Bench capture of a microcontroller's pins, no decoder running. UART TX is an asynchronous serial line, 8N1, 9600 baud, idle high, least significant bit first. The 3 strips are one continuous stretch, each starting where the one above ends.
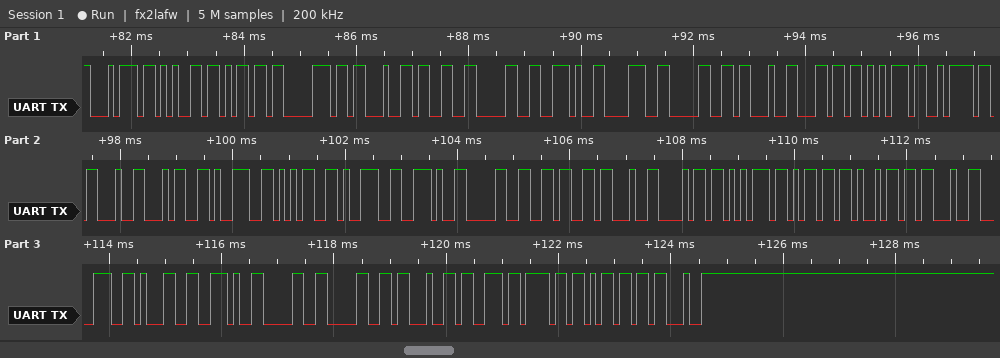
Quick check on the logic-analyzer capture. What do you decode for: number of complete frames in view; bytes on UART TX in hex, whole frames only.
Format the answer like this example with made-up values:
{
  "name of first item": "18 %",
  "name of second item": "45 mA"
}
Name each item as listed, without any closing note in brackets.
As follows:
{
  "number of complete frames in view": "38",
  "bytes on UART TX in hex, whole frames only": "0x74 0x65 0x6D 0x70 0x23 0x33 0x30 0x2E 0x38 0x30 0x23 0x6C 0x75 0x7A 0x23 0x34 0x39 0x35 0x39 0x2E 0x30 0x36 0x23 0x68 0x75 0x6D 0x69 0x23 0x38 0x31 0x2E 0x30 0x30 0x23 0x73 0x6F 0x6D 0x23"
}
